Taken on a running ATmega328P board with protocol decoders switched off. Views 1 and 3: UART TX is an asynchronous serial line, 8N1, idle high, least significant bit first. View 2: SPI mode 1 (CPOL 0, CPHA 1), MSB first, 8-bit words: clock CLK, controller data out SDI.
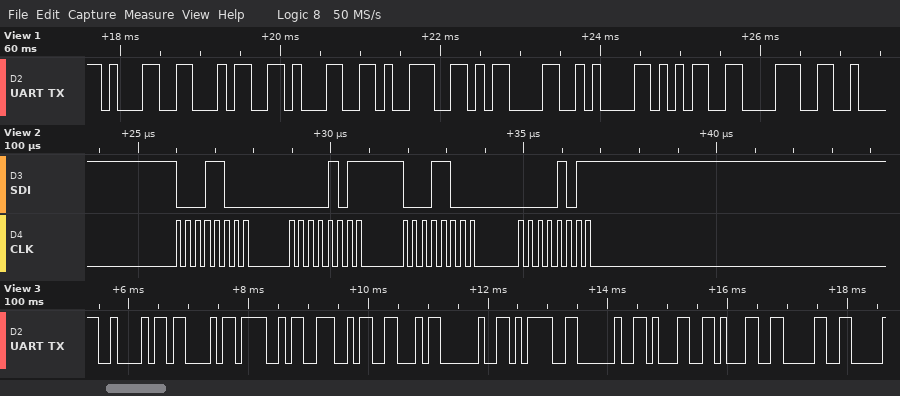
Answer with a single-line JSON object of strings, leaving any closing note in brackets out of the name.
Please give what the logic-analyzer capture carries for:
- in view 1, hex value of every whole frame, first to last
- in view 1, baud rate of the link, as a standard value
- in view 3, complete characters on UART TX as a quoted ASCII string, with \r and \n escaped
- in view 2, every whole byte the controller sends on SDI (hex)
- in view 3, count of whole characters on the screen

{"in view 1, hex value of every whole frame, first to last": "0x31 0x34 0x31 0x39 0x0D 0x0A 0x35 0x38", "in view 1, baud rate of the link, as a standard value": "9600 baud", "in view 3, complete characters on UART TX as a quoted ASCII string, with \\r and \\n escaped": "\"BCONF = 110\"", "in view 2, every whole byte the controller sends on SDI": "0x18 0x0B 0x18 0x0B", "in view 3, count of whole characters on the screen": "11"}
